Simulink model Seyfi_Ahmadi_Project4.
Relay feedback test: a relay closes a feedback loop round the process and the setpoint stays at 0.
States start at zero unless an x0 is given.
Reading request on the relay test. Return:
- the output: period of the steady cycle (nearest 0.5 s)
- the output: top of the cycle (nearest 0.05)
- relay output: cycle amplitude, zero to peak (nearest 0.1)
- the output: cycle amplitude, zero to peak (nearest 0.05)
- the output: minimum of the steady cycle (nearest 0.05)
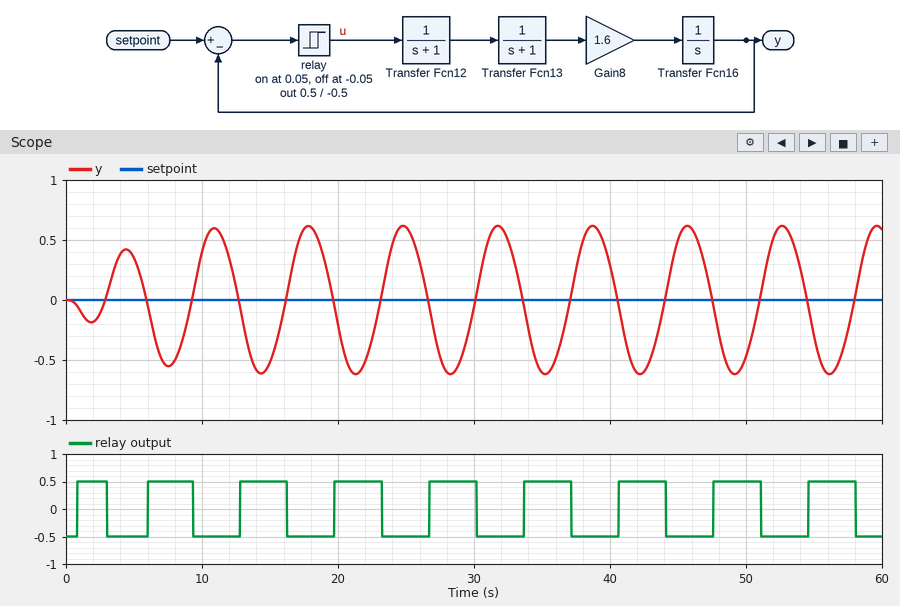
7.0 s
0.60
0.5
0.60
-0.60
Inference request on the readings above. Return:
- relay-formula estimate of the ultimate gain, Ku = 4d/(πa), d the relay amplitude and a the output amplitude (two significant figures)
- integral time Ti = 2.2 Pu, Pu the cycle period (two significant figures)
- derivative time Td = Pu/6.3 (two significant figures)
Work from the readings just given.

1.1
15 s
1.1 s
